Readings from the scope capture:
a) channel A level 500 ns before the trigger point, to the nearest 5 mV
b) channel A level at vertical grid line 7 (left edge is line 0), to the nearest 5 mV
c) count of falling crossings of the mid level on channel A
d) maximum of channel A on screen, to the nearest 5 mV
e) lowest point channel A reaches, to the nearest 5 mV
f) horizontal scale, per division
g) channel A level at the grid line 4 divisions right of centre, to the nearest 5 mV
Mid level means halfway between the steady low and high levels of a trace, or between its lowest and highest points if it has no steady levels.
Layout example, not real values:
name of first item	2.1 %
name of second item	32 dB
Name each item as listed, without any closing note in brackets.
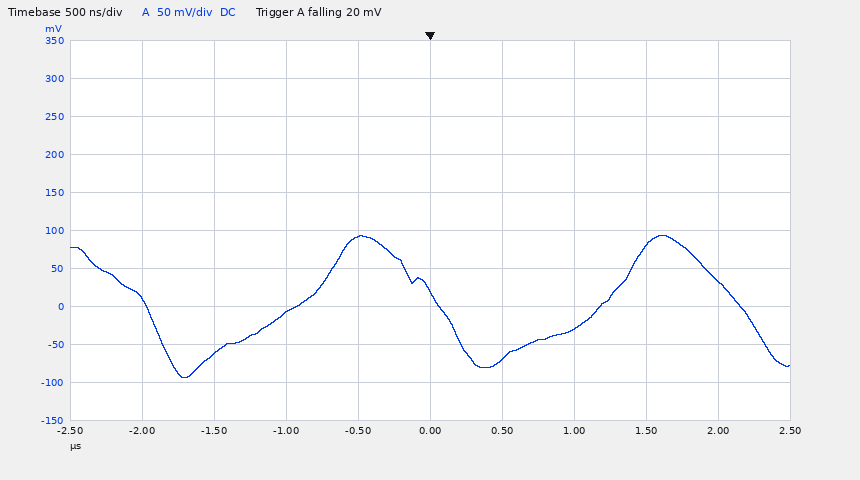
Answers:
channel A level 500 ns before the trigger point, to the nearest 5 mV	90 mV
channel A level at vertical grid line 7 (left edge is line 0), to the nearest 5 mV	-30 mV
count of falling crossings of the mid level on channel A	3
maximum of channel A on screen, to the nearest 5 mV	95 mV
lowest point channel A reaches, to the nearest 5 mV	-95 mV
horizontal scale, per division	500 ns
channel A level at the grid line 4 divisions right of centre, to the nearest 5 mV	35 mV
